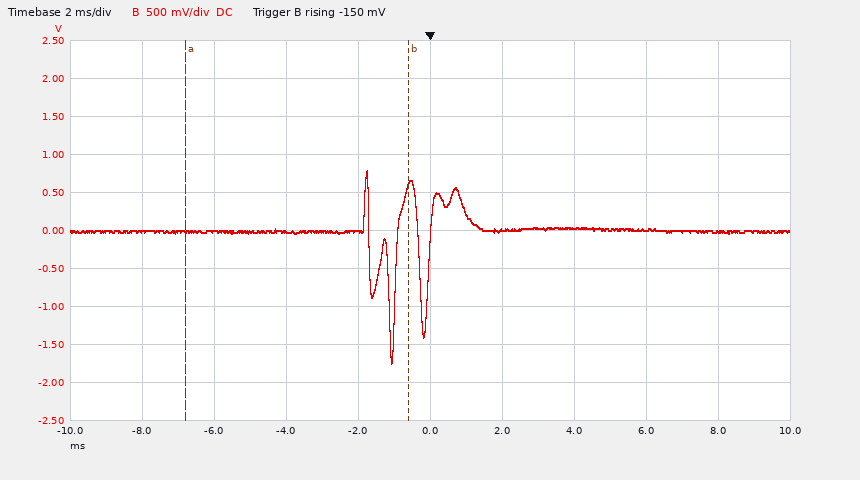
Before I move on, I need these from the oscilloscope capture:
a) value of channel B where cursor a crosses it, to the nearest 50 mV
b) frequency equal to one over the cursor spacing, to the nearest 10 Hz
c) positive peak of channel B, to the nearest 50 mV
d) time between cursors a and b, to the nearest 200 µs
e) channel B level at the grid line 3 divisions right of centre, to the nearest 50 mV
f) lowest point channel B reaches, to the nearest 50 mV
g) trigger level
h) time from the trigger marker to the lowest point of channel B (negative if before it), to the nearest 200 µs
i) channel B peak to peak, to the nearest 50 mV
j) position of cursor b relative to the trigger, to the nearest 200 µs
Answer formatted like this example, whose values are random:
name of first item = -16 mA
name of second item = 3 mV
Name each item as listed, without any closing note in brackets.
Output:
value of channel B where cursor a crosses it, to the nearest 50 mV = 0 mV
frequency equal to one over the cursor spacing, to the nearest 10 Hz = 160 Hz
positive peak of channel B, to the nearest 50 mV = 800 mV
time between cursors a and b, to the nearest 200 µs = 6.2 ms
channel B level at the grid line 3 divisions right of centre, to the nearest 50 mV = 0 mV
lowest point channel B reaches, to the nearest 50 mV = -1.75 V
trigger level = -150 mV
time from the trigger marker to the lowest point of channel B (negative if before it), to the nearest 200 µs = -1.0 ms
channel B peak to peak, to the nearest 50 mV = 2.55 V
position of cursor b relative to the trigger, to the nearest 200 µs = -600 µs
